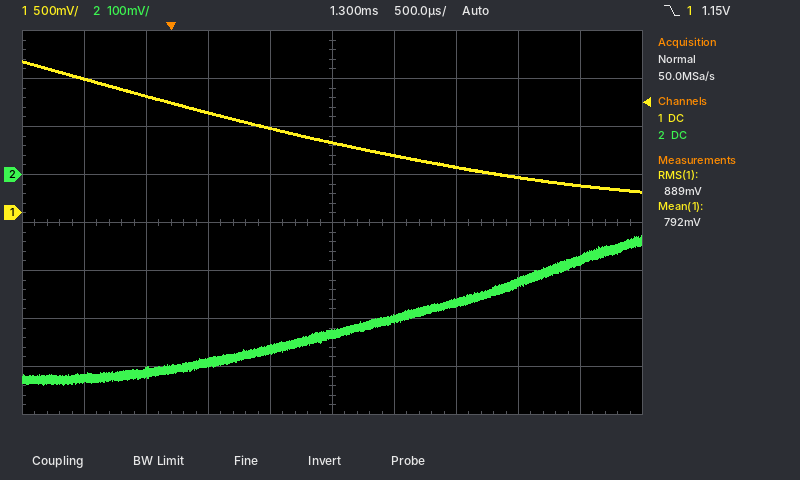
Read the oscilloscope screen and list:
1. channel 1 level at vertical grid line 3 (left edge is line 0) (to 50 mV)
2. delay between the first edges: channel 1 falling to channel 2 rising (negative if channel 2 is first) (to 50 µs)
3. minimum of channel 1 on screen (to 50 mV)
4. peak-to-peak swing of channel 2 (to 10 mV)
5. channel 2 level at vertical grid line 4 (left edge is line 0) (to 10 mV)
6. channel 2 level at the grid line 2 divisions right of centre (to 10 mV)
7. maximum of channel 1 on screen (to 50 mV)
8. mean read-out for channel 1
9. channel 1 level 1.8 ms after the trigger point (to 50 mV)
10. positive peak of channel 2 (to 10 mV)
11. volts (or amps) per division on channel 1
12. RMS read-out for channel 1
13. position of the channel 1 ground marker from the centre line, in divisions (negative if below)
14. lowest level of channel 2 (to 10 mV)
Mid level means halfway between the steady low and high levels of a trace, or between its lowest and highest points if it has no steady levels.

1.05 V
+1.30 ms
200 mV
310 mV
-360 mV
-270 mV
1.60 V
792 mV
600 mV
-130 mV
500 mV
889 mV
+0.2 div
-440 mV
